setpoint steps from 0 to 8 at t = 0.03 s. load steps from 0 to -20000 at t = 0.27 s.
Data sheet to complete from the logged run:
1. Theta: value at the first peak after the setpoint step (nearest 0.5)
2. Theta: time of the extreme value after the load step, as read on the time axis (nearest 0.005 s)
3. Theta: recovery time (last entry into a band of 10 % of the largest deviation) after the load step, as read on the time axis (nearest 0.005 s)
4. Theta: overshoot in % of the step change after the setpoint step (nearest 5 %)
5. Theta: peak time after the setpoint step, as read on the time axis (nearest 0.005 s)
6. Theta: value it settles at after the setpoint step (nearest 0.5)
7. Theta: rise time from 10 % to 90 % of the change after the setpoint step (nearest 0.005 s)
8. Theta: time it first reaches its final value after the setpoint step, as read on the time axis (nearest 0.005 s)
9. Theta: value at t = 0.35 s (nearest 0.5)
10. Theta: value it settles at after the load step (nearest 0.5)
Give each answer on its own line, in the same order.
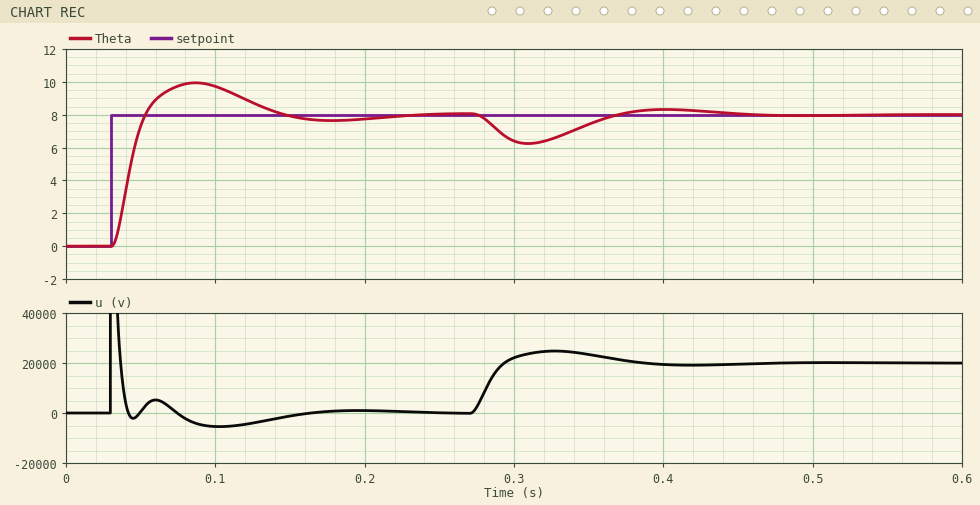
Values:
10.0
0.310 s
0.430 s
25 %
0.085 s
8.0
0.015 s
0.055 s
7.5
8.0
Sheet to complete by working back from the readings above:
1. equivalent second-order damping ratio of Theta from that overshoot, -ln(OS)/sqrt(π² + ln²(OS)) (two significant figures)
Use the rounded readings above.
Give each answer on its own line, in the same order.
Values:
0.40
